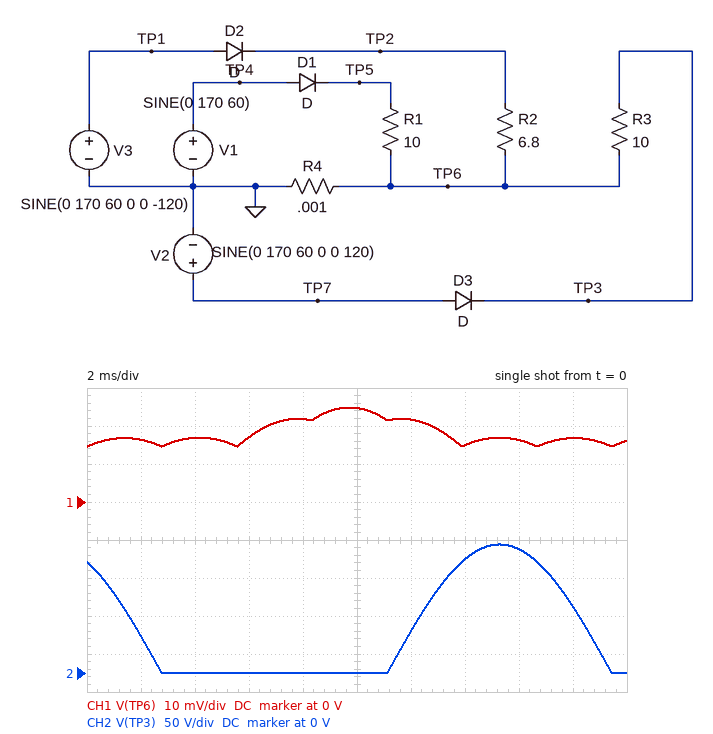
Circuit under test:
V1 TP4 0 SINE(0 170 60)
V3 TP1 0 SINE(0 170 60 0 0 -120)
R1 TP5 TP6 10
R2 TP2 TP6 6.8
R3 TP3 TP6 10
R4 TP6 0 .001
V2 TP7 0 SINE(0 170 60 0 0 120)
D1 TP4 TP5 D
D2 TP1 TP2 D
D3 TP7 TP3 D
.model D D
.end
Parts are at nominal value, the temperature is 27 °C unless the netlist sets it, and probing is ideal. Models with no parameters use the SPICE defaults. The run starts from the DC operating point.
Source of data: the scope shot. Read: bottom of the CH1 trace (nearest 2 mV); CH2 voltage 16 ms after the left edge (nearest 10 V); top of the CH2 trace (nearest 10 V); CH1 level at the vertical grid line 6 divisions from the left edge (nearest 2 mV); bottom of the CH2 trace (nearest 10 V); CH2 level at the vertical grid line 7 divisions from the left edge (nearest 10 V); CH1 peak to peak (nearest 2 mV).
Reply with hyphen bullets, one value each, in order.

- 14 mV
- 160 V
- 170 V
- 22 mV
- 0 V
- 150 V
- 10 mV
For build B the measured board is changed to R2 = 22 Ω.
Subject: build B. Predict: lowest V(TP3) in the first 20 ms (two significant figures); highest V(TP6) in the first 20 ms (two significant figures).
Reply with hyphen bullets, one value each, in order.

- 6.6 mV
- 17 mV
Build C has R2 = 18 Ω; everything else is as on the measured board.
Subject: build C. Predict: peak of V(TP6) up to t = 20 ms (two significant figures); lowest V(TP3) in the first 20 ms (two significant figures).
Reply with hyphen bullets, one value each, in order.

- 17 mV
- 8.1 mV
